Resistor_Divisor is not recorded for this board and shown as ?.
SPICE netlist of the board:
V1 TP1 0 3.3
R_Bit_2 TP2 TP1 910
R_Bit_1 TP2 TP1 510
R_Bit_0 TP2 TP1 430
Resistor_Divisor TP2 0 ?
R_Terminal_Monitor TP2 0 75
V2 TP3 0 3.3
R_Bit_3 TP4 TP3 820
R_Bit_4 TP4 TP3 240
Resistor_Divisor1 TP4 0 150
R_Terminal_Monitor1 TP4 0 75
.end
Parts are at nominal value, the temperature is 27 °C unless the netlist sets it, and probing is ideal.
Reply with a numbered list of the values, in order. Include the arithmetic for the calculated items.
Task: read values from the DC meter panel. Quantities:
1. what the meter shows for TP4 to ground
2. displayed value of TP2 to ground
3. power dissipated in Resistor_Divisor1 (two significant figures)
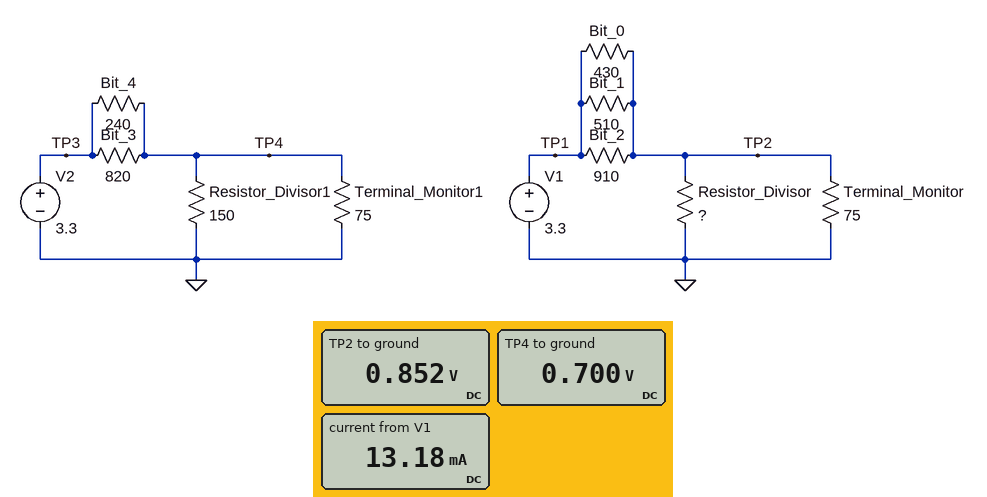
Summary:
1. 0.700 V
2. 0.852 V
3. (700 mV)^2 / 150 Ω = 3.3 mW
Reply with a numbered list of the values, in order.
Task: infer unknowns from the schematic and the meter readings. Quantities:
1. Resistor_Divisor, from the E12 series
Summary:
1. 470 Ω
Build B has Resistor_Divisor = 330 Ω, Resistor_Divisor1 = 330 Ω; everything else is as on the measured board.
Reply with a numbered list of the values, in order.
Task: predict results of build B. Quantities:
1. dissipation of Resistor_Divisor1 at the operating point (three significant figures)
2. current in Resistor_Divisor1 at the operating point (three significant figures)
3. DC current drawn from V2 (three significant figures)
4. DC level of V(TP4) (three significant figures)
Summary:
1. 2.02 mW
2. 2.48 mA
3. 13.4 mA
4. 817 mV
